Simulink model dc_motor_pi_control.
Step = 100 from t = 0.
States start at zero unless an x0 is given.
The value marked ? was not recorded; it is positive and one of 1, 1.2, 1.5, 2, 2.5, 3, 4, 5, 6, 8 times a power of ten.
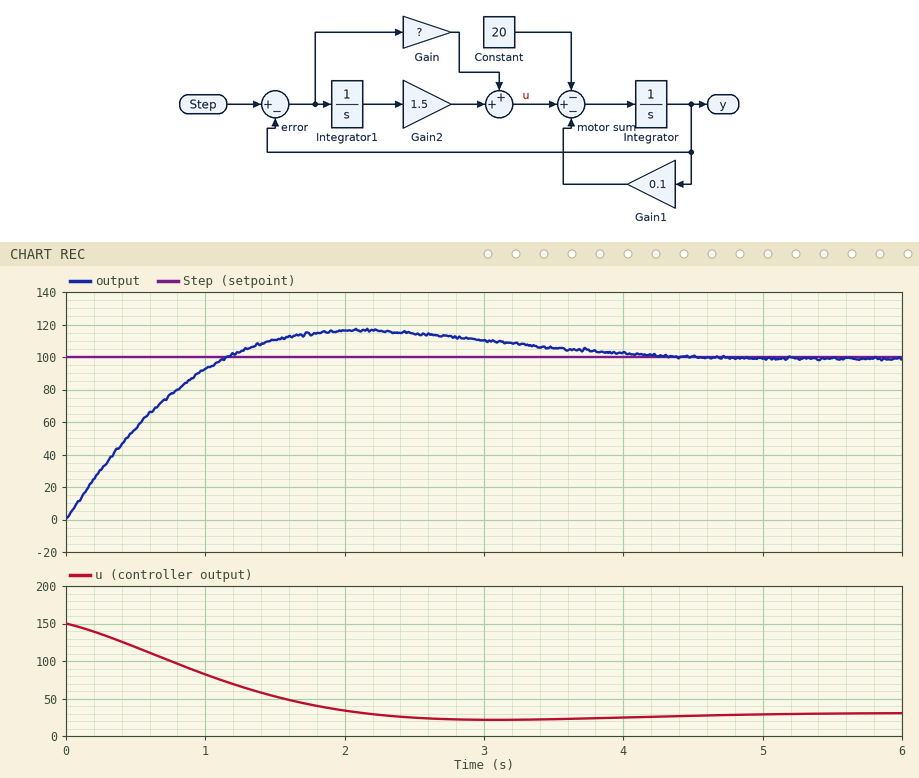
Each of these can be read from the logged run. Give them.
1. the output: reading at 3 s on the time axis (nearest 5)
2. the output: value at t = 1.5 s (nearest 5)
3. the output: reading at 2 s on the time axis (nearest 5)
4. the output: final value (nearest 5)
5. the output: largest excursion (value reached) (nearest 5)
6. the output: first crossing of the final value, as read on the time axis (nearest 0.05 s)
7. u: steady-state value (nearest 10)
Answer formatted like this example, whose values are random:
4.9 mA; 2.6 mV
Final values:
110; 110; 115; 100; 115; 1.15 s; 30
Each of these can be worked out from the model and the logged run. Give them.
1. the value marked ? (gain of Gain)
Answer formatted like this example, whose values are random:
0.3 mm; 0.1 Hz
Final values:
1.5
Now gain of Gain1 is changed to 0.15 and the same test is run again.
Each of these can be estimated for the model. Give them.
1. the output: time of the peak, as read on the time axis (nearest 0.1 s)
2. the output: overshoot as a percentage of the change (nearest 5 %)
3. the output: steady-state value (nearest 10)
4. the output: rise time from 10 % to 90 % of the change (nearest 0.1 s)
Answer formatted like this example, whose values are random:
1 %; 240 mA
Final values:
2.1 s; 15 %; 100; 0.9 s
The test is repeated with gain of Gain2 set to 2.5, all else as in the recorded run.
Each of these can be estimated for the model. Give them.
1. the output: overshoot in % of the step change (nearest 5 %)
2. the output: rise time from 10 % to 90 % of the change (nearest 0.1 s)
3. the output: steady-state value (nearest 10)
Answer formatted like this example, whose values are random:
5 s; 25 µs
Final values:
25 %; 0.7 s; 100
